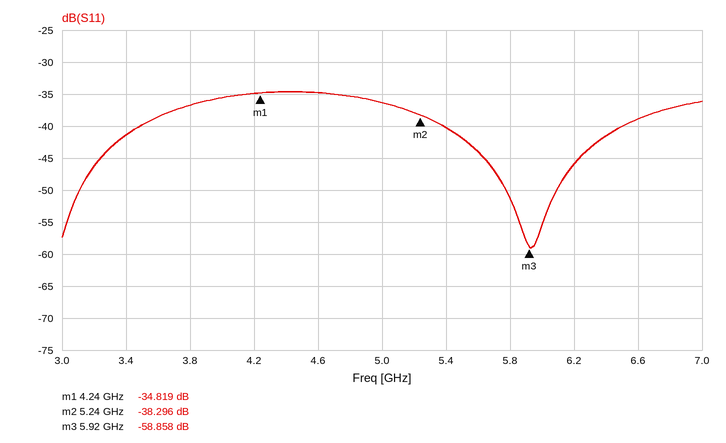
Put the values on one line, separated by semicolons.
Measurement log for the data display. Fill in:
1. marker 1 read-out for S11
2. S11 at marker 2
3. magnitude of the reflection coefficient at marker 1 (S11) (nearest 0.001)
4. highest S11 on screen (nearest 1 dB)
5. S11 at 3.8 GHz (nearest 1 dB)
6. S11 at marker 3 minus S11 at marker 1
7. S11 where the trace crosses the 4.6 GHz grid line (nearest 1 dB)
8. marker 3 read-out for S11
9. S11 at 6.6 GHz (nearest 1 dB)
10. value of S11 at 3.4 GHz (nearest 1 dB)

-34.819 dB; -38.296 dB; 0.018; -35 dB; -37 dB; -24.039 dB; -35 dB; -58.858 dB; -39 dB; -41 dB
